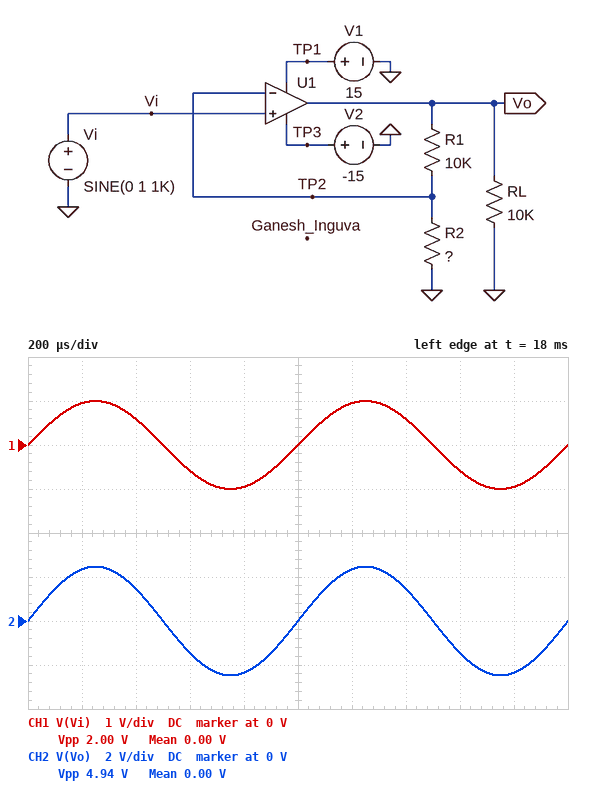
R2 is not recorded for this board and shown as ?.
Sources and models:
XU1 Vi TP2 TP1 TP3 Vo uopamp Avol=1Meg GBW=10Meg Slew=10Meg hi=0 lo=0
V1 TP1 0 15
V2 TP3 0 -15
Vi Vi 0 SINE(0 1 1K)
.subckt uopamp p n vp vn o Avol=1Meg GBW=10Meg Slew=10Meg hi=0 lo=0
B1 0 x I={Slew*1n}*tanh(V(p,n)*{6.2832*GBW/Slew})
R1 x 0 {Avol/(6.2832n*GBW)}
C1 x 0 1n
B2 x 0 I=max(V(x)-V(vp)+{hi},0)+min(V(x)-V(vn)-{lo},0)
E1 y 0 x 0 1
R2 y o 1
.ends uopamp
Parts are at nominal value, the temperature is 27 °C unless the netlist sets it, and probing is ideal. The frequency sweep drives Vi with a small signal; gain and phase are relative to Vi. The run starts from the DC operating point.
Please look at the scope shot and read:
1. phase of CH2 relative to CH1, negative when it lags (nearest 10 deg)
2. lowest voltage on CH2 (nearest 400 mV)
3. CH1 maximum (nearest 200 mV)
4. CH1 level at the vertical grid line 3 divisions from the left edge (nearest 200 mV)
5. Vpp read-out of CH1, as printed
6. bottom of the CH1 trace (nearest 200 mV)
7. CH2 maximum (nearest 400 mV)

0 deg
-2.4 V
1.0 V
-600 mV
2.00 V
-1.0 V
2.4 V
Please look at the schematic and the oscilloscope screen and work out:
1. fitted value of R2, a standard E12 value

6.8 kΩ
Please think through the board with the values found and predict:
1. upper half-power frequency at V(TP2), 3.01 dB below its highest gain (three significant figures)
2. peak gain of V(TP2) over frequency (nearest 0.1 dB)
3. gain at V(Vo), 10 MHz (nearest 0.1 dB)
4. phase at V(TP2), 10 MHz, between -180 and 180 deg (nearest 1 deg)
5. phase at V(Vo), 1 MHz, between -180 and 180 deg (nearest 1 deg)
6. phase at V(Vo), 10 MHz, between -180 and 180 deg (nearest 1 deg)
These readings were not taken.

4.05 MHz
0 dB
-0.7 dB
-68 deg
-14 deg
-68 deg
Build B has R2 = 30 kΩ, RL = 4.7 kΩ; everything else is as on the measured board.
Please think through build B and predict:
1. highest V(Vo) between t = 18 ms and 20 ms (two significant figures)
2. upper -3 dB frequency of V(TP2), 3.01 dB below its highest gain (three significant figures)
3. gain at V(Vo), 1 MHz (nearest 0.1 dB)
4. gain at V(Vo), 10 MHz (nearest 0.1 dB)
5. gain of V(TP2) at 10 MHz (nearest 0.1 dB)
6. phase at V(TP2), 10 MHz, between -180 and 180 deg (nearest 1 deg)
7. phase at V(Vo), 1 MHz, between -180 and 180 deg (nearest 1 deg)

1.3 V
7.50 MHz
2.4 dB
-1.9 dB
-4.4 dB
-53 deg
-8 deg
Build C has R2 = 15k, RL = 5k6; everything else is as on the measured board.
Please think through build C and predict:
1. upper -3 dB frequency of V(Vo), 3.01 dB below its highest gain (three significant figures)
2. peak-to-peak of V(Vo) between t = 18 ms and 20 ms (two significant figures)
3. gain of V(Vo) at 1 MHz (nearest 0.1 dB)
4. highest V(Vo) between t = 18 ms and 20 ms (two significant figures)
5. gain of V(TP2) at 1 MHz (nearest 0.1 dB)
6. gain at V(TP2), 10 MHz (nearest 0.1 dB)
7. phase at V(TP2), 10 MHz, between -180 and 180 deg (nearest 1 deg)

6.00 MHz
3.3 V
4.3 dB
1.7 V
-0.1 dB
-5.8 dB
-59 deg
